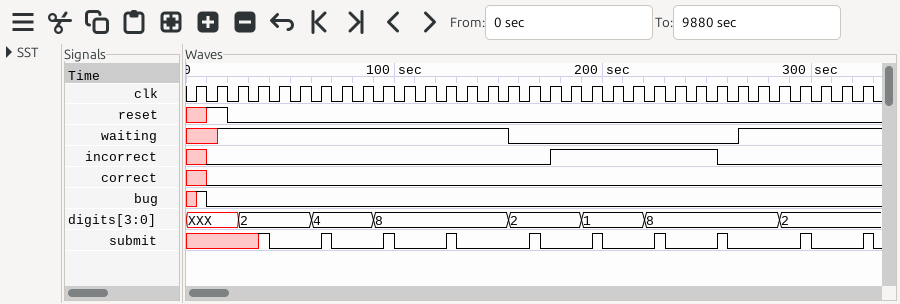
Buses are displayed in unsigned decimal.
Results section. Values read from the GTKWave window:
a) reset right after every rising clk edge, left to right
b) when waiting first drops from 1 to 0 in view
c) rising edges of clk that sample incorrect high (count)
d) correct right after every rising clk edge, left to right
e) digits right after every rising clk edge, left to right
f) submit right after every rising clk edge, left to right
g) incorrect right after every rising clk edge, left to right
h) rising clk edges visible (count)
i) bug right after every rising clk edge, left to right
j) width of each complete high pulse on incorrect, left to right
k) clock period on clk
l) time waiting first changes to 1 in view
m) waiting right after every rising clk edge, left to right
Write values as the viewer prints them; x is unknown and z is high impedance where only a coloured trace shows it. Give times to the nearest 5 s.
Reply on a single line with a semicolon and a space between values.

x 1 0 0 0 0 0 0 0 0 0 0 0 0 0 0 0 0 0 0 0 0 0 0 0 0 0 0 0 0 0 0 0; 155 s; 8; x 0 0 0 0 0 0 0 0 0 0 0 0 0 0 0 0 0 0 0 0 0 0 0 0 0 0 0 0 0 0 0 0; XXX, XXX, 2, 2, 2, 2, 4, 4, 4, 8, 8, 8, 8, 8, 8, 2, 2, 2, 2, 1, 1, 1, 8, 8, 8, 8, 8, 8, 2, 2, 2, 2, 2; x x x 1 0 0 1 0 0 1 0 0 1 0 0 0 1 0 0 1 0 0 1 0 0 1 0 0 0 1 0 0 1; x 0 0 0 0 0 0 0 0 0 0 0 0 0 0 0 0 1 1 1 1 1 1 1 1 0 0 0 0 0 0 0 0; 33; 1 0 0 0 0 0 0 0 0 0 0 0 0 0 0 0 0 0 0 0 0 0 0 0 0 0 0 0 0 0 0 0 0; 80 s; 10 s; 15 s; x 1 1 1 1 1 1 1 1 1 1 1 1 1 1 0 0 0 0 0 0 0 0 0 0 0 1 1 1 1 1 1 1
